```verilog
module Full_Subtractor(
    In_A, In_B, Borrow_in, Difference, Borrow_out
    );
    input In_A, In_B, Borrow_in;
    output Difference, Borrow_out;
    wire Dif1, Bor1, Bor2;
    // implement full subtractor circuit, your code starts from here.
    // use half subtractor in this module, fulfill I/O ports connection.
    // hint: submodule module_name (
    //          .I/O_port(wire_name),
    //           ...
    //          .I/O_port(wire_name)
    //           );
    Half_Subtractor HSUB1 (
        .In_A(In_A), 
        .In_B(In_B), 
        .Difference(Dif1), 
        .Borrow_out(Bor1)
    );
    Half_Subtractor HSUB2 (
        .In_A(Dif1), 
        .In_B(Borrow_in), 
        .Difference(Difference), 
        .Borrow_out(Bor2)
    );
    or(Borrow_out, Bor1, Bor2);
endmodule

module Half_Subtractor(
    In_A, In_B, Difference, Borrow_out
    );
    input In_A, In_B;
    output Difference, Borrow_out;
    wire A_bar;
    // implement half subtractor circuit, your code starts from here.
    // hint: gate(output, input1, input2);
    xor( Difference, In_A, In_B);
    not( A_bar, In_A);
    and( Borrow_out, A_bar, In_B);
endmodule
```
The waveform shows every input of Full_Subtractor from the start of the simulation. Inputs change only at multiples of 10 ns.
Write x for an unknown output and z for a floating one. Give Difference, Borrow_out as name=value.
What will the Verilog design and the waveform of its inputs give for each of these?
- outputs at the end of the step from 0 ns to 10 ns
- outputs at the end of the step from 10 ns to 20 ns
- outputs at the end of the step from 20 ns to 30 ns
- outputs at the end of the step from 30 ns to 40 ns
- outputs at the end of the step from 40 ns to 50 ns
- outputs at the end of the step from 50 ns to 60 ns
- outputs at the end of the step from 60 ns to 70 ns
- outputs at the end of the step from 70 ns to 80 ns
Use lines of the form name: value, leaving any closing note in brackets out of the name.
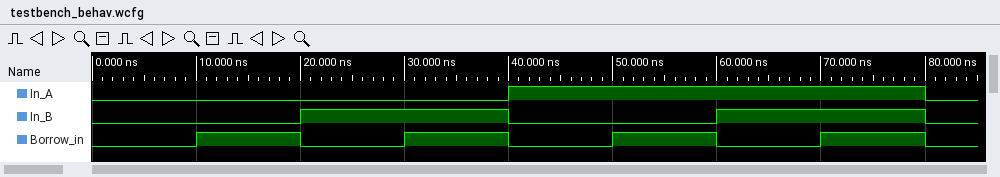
outputs at the end of the step from 0 ns to 10 ns: Difference=0, Borrow_out=0
outputs at the end of the step from 10 ns to 20 ns: Difference=1, Borrow_out=1
outputs at the end of the step from 20 ns to 30 ns: Difference=1, Borrow_out=1
outputs at the end of the step from 30 ns to 40 ns: Difference=0, Borrow_out=1
outputs at the end of the step from 40 ns to 50 ns: Difference=1, Borrow_out=0
outputs at the end of the step from 50 ns to 60 ns: Difference=0, Borrow_out=0
outputs at the end of the step from 60 ns to 70 ns: Difference=0, Borrow_out=0
outputs at the end of the step from 70 ns to 80 ns: Difference=1, Borrow_out=1
